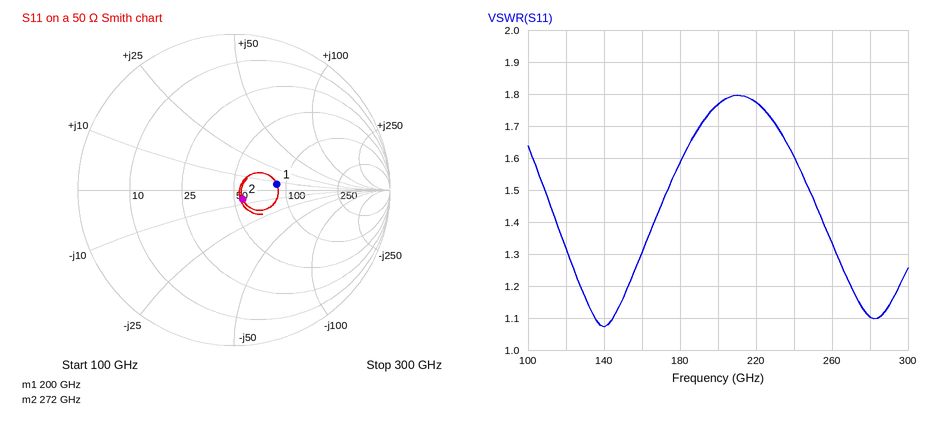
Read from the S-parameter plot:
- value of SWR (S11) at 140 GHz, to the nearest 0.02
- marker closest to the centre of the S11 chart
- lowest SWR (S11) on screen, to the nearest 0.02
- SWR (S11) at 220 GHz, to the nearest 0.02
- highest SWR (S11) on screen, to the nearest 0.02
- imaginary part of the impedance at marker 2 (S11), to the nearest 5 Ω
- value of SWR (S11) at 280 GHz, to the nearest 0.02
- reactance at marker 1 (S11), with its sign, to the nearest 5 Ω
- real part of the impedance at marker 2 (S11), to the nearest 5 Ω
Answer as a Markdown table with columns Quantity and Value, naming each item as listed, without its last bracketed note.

| Quantity | Value |
|---|---|
| value of SWR (S11) at 140 GHz, to the nearest 0.02 | 1.08 |
| marker closest to the centre of the S11 chart | marker 2 |
| lowest SWR (S11) on screen, to the nearest 0.02 | 1.08 |
| SWR (S11) at 220 GHz, to the nearest 0.02 | 1.78 |
| highest SWR (S11) on screen, to the nearest 0.02 | 1.80 |
| imaginary part of the impedance at marker 2 (S11), to the nearest 5 Ω | -5 Ω |
| value of SWR (S11) at 280 GHz, to the nearest 0.02 | 1.10 |
| reactance at marker 1 (S11), with its sign, to the nearest 5 Ω | +5 Ω |
| real part of the impedance at marker 2 (S11), to the nearest 5 Ω | 55 Ω |
